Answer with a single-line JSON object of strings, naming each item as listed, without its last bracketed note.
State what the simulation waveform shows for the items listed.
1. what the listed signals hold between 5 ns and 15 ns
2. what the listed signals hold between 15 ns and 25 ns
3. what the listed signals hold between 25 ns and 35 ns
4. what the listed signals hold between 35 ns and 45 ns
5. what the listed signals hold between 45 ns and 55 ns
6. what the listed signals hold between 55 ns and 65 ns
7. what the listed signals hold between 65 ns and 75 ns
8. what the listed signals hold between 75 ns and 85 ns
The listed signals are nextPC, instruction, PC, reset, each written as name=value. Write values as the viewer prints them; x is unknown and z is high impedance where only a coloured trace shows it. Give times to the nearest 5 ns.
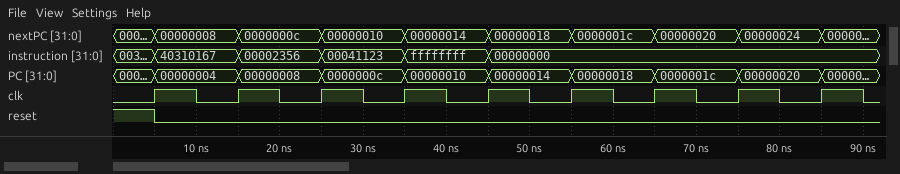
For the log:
{"what the listed signals hold between 5 ns and 15 ns": "nextPC=00000008, instruction=40310167, PC=00000004, reset=0", "what the listed signals hold between 15 ns and 25 ns": "nextPC=0000000c, instruction=00002356, PC=00000008, reset=0", "what the listed signals hold between 25 ns and 35 ns": "nextPC=00000010, instruction=00041123, PC=0000000c, reset=0", "what the listed signals hold between 35 ns and 45 ns": "nextPC=00000014, instruction=ffffffff, PC=00000010, reset=0", "what the listed signals hold between 45 ns and 55 ns": "nextPC=00000018, instruction=00000000, PC=00000014, reset=0", "what the listed signals hold between 55 ns and 65 ns": "nextPC=0000001c, instruction=00000000, PC=00000018, reset=0", "what the listed signals hold between 65 ns and 75 ns": "nextPC=00000020, instruction=00000000, PC=0000001c, reset=0", "what the listed signals hold between 75 ns and 85 ns": "nextPC=00000024, instruction=00000000, PC=00000020, reset=0"}
